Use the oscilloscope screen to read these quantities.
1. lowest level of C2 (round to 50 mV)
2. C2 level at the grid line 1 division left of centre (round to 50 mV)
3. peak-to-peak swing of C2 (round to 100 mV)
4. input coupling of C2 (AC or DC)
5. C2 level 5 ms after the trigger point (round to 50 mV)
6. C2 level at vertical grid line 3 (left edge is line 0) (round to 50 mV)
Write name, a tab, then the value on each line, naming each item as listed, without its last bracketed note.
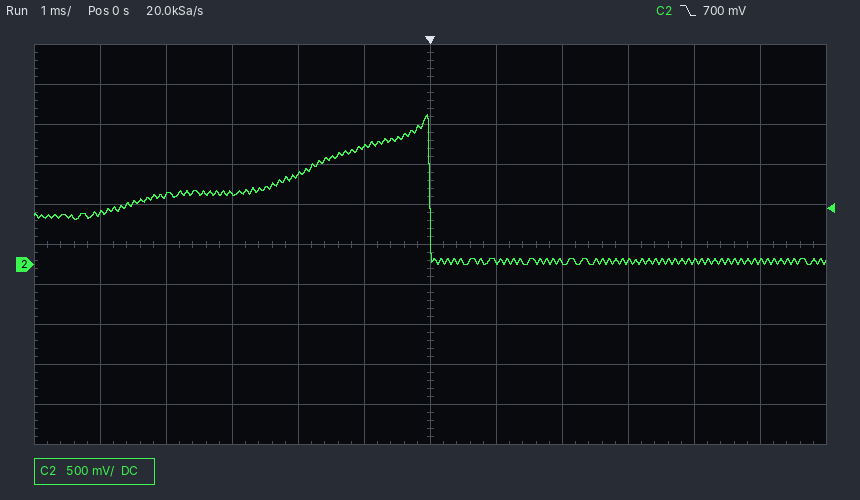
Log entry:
lowest level of C2	0 mV
C2 level at the grid line 1 division left of centre	1.45 V
peak-to-peak swing of C2	1.90 V
input coupling of C2	DC
C2 level 5 ms after the trigger point	50 mV
C2 level at vertical grid line 3 (left edge is line 0)	900 mV
